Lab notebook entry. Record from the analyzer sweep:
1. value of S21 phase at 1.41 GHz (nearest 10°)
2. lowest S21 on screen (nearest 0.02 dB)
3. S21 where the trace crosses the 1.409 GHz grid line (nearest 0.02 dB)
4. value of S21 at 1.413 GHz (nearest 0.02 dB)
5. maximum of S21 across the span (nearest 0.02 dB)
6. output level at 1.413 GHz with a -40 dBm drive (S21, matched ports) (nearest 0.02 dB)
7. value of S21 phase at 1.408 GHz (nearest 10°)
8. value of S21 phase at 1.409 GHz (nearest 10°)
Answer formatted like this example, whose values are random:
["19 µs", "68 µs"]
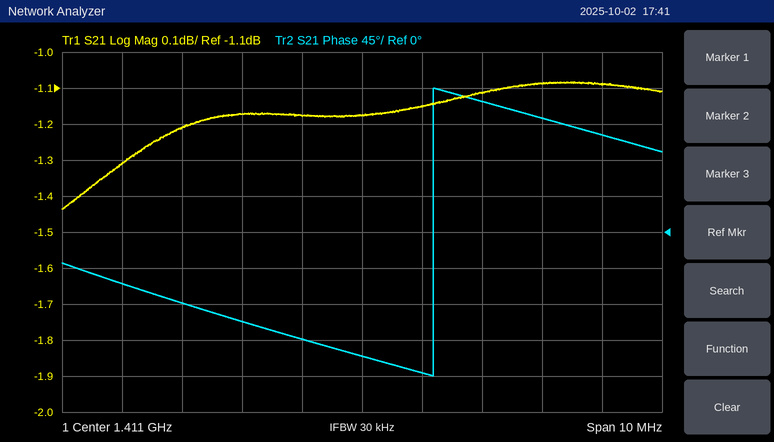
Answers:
["-130°", "-1.44 dB", "-1.18 dB", "-1.12 dB", "-1.08 dB", "-41.12 dBm", "-90°", "-110°"]
